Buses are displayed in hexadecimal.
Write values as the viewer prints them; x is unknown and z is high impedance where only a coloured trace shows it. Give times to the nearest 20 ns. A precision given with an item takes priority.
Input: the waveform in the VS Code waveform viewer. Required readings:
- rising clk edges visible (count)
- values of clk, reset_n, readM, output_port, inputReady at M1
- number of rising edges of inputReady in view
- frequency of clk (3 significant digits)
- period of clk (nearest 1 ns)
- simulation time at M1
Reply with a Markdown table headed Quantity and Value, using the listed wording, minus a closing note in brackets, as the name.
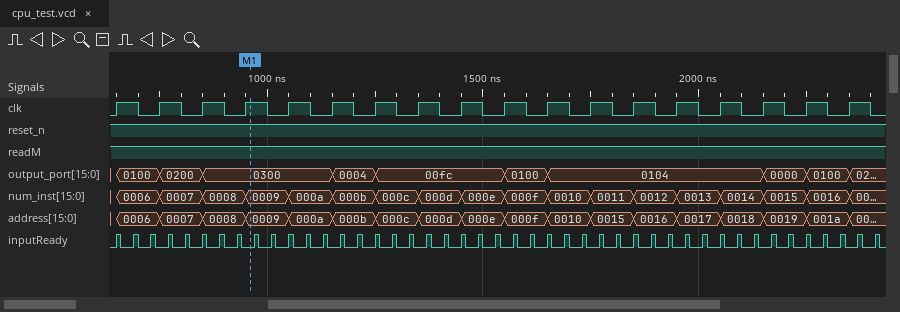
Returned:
| Quantity | Value |
|---|---|
| rising clk edges visible | 18 |
| values of clk, reset_n, readM, output_port, inputReady at M1 | clk=1, reset_n=1, readM=1, output_port=0300, inputReady=0 |
| number of rising edges of inputReady in view | 45 |
| frequency of clk | 10.0 MHz |
| period of clk | 100 ns |
| simulation time at M1 | 960 ns |
